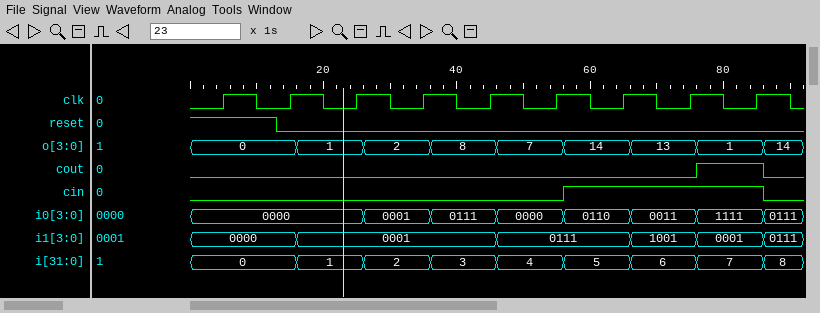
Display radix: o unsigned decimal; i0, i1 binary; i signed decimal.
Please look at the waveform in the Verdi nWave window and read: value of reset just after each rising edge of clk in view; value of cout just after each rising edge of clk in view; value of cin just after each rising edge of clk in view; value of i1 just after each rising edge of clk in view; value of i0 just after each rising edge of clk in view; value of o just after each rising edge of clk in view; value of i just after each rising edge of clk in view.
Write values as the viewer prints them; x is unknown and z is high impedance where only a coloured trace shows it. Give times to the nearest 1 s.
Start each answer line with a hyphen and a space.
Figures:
- 1 0 0 0 0 0 0 0 0
- 0 0 0 0 0 0 0 0 1
- 0 0 0 0 0 0 1 1 1
- 0000, 0000, 0001, 0001, 0001, 0111, 0111, 1001, 0001
- 0000, 0000, 0000, 0001, 0111, 0000, 0110, 0011, 1111
- 0, 0, 1, 2, 8, 7, 14, 13, 1
- 0, 0, 1, 2, 3, 4, 5, 6, 7
